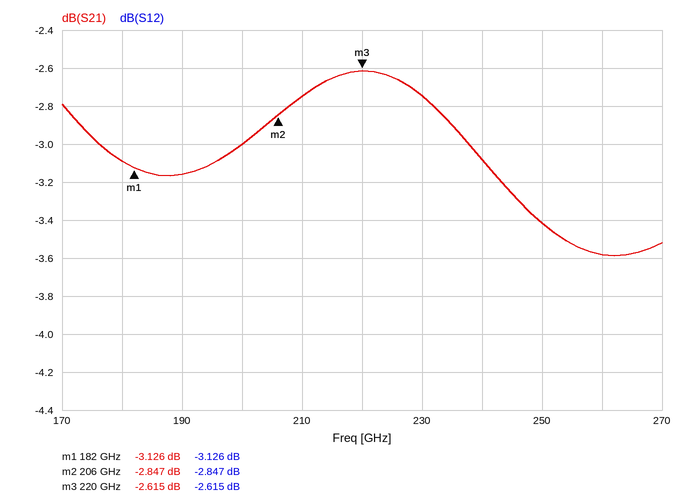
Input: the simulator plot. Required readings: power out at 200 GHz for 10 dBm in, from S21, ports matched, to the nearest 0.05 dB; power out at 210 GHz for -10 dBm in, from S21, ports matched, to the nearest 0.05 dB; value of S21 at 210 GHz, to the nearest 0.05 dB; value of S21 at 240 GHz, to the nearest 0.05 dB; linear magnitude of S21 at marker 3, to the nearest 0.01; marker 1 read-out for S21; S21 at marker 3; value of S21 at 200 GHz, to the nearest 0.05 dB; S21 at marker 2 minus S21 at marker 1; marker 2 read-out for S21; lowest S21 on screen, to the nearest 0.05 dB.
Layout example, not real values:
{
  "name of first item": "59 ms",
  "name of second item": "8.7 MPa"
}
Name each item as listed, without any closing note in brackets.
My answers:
{
  "power out at 200 GHz for 10 dBm in, from S21, ports matched, to the nearest 0.05 dB": "7.00 dBm",
  "power out at 210 GHz for -10 dBm in, from S21, ports matched, to the nearest 0.05 dB": "-12.75 dBm",
  "value of S21 at 210 GHz, to the nearest 0.05 dB": "-2.75 dB",
  "value of S21 at 240 GHz, to the nearest 0.05 dB": "-3.10 dB",
  "linear magnitude of S21 at marker 3, to the nearest 0.01": "0.74",
  "marker 1 read-out for S21": "-3.126 dB",
  "S21 at marker 3": "-2.615 dB",
  "value of S21 at 200 GHz, to the nearest 0.05 dB": "-3.00 dB",
  "S21 at marker 2 minus S21 at marker 1": "0.279 dB",
  "marker 2 read-out for S21": "-2.847 dB",
  "lowest S21 on screen, to the nearest 0.05 dB": "-3.60 dB"
}
